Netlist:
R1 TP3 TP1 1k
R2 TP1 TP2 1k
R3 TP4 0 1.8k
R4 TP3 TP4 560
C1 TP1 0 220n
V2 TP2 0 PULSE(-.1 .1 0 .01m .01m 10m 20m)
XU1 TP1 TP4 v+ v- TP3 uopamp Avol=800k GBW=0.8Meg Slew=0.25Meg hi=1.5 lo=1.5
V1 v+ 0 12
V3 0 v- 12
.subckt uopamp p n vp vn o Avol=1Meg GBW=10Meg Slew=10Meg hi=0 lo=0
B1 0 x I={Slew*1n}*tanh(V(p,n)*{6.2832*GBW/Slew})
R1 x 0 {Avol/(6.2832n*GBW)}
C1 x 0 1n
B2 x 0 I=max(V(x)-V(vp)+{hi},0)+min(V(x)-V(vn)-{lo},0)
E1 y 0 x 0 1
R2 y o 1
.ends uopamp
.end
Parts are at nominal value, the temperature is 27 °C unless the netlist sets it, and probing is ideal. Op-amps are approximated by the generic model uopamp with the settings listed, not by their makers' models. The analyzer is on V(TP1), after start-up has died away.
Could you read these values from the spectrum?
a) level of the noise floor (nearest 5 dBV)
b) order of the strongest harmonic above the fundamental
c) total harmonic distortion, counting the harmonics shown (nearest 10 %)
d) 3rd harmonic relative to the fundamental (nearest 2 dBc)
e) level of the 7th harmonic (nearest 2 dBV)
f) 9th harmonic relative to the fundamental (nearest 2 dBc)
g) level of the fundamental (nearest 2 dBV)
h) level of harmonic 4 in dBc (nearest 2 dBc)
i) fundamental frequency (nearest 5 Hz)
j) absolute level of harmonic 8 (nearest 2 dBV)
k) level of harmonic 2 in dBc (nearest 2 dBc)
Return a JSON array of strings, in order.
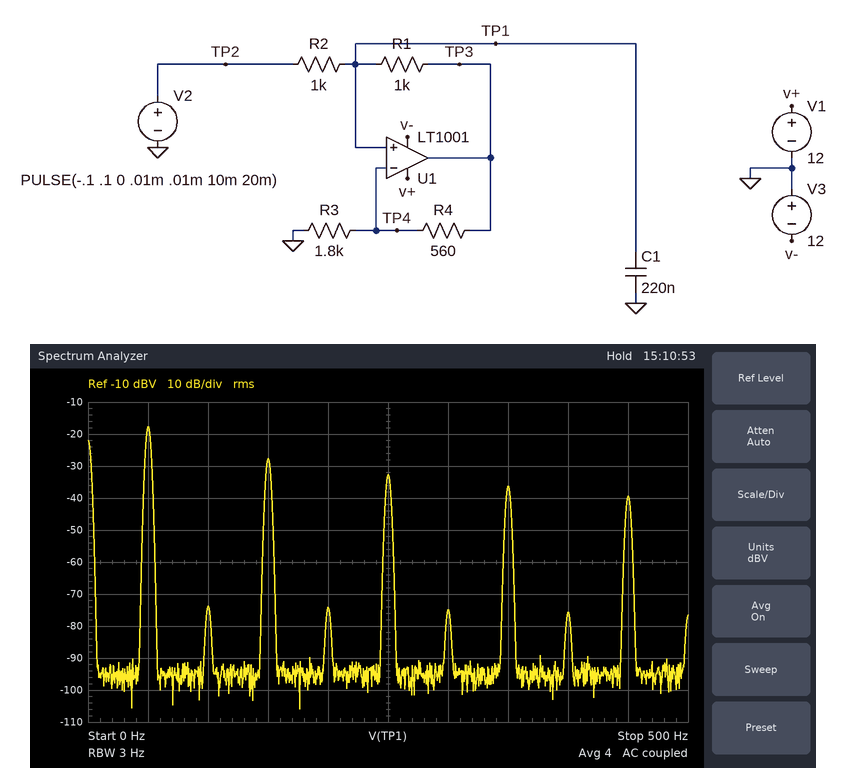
["-95 dBV", "3", "40 %", "-10 dBc", "-36 dBV", "-22 dBc", "-18 dBV", "-56 dBc", "50 Hz", "-76 dBV", "-56 dBc"]
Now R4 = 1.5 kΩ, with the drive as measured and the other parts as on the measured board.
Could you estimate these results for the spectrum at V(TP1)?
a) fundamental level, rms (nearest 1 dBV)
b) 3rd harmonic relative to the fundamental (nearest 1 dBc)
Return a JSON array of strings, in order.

["-6 dBV", "-13 dBc"]
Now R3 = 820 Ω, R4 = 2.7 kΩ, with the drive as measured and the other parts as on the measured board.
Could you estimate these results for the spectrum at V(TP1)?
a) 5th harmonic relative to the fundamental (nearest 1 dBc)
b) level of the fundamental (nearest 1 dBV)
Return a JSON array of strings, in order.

["-14 dBc", "-27 dBV"]
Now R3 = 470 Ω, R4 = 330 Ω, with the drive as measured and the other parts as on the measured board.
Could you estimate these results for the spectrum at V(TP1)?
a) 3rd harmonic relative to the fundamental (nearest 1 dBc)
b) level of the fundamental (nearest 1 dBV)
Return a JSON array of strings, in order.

["-11 dBc", "-11 dBV"]
